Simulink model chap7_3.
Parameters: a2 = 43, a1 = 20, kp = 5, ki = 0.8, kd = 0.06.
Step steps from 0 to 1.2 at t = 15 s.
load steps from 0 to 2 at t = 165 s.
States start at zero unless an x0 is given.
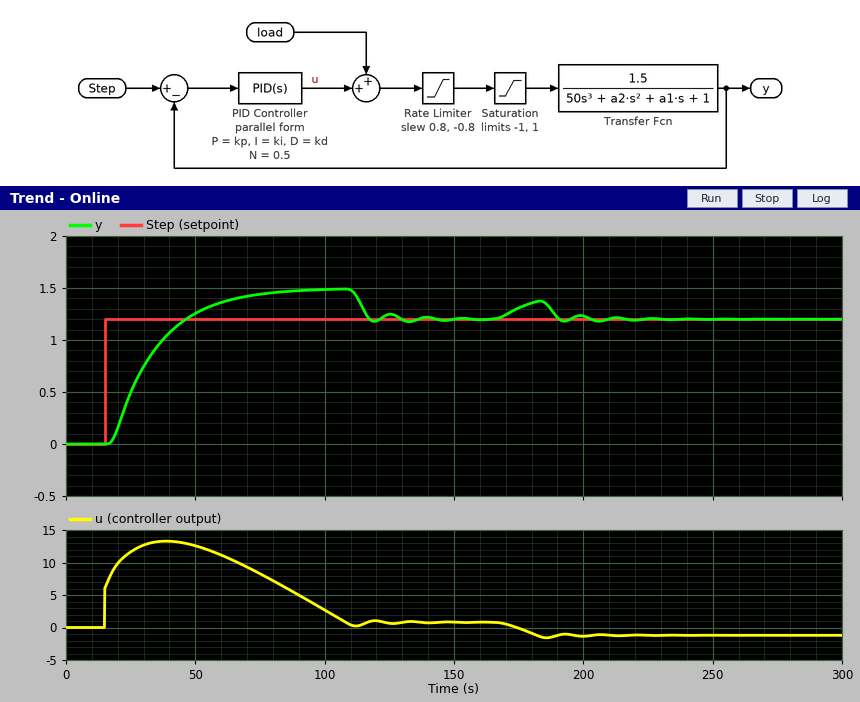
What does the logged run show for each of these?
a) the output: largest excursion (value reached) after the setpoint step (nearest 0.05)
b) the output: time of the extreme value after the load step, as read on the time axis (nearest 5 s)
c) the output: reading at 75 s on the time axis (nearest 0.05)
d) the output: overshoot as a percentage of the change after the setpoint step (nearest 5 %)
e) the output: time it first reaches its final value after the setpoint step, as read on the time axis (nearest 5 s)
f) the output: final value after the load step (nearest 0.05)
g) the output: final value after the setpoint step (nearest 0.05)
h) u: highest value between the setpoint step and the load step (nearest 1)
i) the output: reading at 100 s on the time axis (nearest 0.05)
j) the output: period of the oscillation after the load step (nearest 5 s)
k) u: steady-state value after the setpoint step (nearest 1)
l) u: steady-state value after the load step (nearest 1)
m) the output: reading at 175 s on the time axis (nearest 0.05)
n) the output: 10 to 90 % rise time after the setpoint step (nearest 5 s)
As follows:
1.50
185 s
1.45
25 %
45 s
1.20
1.20
13
1.50
15 s
1
-1
1.30
20 s
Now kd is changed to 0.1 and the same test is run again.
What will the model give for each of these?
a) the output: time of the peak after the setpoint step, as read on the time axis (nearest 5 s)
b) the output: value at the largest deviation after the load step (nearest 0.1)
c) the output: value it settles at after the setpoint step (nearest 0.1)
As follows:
110 s
1.4
1.2
